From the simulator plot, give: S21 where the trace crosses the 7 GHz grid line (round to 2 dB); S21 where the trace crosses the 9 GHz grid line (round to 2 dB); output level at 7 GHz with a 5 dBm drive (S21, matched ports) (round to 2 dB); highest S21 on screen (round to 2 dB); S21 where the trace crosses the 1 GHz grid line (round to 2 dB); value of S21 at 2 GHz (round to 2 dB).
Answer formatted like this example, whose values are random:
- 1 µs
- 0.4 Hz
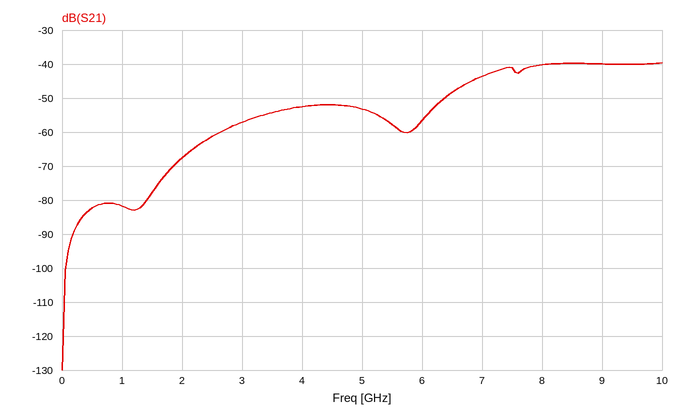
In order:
- -44 dB
- -40 dB
- -38 dBm
- -40 dB
- -82 dB
- -68 dB
